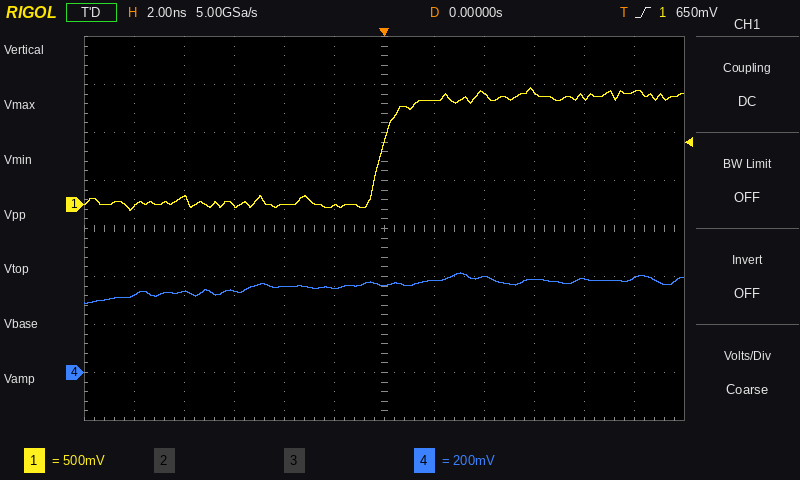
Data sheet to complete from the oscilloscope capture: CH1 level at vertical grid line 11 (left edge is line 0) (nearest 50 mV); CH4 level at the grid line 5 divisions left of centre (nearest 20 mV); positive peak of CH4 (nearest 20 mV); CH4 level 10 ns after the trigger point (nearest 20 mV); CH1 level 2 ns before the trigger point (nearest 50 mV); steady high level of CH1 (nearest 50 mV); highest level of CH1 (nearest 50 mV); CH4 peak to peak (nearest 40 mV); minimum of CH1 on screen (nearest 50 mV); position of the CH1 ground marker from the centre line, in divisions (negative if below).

1.15 V
320 mV
420 mV
400 mV
0 mV
1.10 V
1.20 V
120 mV
-50 mV
+0.5 div
